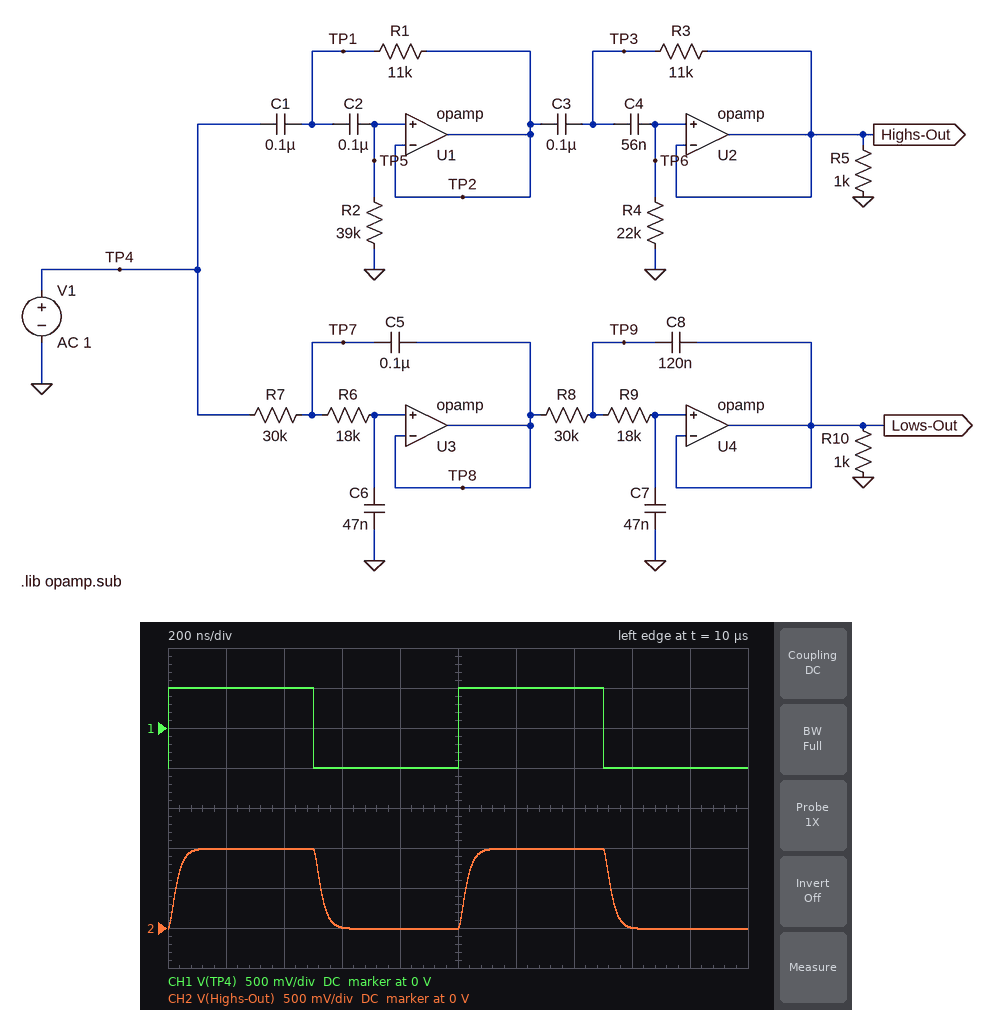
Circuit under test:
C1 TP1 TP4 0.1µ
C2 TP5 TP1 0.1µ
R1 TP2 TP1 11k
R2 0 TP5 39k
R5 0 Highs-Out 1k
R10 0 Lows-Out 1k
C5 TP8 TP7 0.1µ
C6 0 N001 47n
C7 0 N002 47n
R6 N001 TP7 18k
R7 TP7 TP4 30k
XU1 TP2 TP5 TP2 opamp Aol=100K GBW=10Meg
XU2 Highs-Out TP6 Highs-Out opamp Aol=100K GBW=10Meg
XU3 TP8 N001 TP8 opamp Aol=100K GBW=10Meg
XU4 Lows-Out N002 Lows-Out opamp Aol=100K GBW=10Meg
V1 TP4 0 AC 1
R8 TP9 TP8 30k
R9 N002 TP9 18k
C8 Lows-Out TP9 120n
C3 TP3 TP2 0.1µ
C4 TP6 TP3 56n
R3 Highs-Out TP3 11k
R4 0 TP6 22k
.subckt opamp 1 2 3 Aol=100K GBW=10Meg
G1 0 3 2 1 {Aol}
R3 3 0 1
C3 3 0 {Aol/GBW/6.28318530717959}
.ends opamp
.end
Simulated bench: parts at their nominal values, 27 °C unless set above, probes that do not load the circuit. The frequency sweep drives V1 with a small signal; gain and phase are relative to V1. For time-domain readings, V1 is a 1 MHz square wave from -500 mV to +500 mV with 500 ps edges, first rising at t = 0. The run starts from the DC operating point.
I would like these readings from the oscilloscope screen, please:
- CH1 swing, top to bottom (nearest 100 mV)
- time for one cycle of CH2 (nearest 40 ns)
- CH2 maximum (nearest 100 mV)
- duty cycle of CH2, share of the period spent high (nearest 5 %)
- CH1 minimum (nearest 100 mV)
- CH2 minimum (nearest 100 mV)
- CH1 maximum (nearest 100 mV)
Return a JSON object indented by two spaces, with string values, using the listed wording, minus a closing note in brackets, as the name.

{
  "CH1 swing, top to bottom": "1.0 V",
  "time for one cycle of CH2": "1.00 µs",
  "CH2 maximum": "1.0 V",
  "duty cycle of CH2, share of the period spent high": "50 %",
  "CH1 minimum": "-500 mV",
  "CH2 minimum": "0 V",
  "CH1 maximum": "500 mV"
}
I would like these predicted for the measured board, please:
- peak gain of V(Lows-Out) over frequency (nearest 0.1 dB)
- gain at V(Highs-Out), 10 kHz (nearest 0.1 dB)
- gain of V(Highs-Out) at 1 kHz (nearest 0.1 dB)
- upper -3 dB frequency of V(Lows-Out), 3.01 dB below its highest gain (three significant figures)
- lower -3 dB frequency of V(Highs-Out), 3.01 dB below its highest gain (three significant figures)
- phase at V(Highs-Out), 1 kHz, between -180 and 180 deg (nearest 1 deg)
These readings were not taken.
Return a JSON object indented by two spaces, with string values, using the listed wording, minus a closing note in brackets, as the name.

{
  "peak gain of V(Lows-Out) over frequency": "0.1 dB",
  "gain at V(Highs-Out), 10 kHz": "0 dB",
  "gain of V(Highs-Out) at 1 kHz": "0 dB",
  "upper -3 dB frequency of V(Lows-Out), 3.01 dB below its highest gain": "81.2 Hz",
  "lower -3 dB frequency of V(Highs-Out), 3.01 dB below its highest gain": "129 Hz",
  "phase at V(Highs-Out), 1 kHz, between -180 and 180 deg": "16 deg"
}
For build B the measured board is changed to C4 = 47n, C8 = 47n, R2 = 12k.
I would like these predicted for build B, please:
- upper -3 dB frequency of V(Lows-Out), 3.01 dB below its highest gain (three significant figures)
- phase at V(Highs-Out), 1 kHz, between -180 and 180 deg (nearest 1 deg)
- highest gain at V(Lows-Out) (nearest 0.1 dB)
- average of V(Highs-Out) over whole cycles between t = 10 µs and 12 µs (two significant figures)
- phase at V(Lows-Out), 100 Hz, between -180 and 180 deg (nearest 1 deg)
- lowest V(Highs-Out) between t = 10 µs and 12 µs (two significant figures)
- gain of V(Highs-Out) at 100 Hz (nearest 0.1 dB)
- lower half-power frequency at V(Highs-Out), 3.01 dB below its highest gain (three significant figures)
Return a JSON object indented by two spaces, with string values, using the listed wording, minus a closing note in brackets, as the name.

{
  "upper -3 dB frequency of V(Lows-Out), 3.01 dB below its highest gain": "70.9 Hz",
  "phase at V(Highs-Out), 1 kHz, between -180 and 180 deg": "28 deg",
  "highest gain at V(Lows-Out)": "0 dB",
  "average of V(Highs-Out) over whole cycles between t = 10 µs and 12 µs": "480 mV",
  "phase at V(Lows-Out), 100 Hz, between -180 and 180 deg": "-160 deg",
  "lowest V(Highs-Out) between t = 10 µs and 12 µs": "-18 mV",
  "gain of V(Highs-Out) at 100 Hz": "-17.2 dB",
  "lower half-power frequency at V(Highs-Out), 3.01 dB below its highest gain": "248 Hz"
}
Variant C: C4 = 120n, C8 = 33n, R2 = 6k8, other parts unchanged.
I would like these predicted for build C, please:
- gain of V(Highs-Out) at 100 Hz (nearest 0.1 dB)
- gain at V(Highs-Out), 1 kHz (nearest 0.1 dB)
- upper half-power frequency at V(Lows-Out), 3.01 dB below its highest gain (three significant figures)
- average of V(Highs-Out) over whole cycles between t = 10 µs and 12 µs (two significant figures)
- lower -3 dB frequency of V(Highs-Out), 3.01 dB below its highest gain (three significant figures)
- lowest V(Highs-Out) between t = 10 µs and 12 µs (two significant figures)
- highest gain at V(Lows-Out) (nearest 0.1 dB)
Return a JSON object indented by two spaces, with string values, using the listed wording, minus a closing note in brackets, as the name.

{
  "gain of V(Highs-Out) at 100 Hz": "-16.9 dB",
  "gain at V(Highs-Out), 1 kHz": "-0.6 dB",
  "upper half-power frequency at V(Lows-Out), 3.01 dB below its highest gain": "67.9 Hz",
  "average of V(Highs-Out) over whole cycles between t = 10 µs and 12 µs": "480 mV",
  "lower -3 dB frequency of V(Highs-Out), 3.01 dB below its highest gain": "400 Hz",
  "lowest V(Highs-Out) between t = 10 µs and 12 µs": "-22 mV",
  "highest gain at V(Lows-Out)": "0 dB"
}
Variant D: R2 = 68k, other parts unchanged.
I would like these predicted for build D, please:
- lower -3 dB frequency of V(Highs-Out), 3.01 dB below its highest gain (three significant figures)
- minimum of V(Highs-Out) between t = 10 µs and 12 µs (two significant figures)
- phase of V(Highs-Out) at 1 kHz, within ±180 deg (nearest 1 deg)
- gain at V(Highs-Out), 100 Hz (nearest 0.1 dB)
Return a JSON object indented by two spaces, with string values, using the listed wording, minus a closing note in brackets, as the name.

{
  "lower -3 dB frequency of V(Highs-Out), 3.01 dB below its highest gain": "125 Hz",
  "minimum of V(Highs-Out) between t = 10 µs and 12 µs": "-9.3 mV",
  "phase of V(Highs-Out) at 1 kHz, within ±180 deg": "14 deg",
  "gain at V(Highs-Out), 100 Hz": "-5.0 dB"
}
